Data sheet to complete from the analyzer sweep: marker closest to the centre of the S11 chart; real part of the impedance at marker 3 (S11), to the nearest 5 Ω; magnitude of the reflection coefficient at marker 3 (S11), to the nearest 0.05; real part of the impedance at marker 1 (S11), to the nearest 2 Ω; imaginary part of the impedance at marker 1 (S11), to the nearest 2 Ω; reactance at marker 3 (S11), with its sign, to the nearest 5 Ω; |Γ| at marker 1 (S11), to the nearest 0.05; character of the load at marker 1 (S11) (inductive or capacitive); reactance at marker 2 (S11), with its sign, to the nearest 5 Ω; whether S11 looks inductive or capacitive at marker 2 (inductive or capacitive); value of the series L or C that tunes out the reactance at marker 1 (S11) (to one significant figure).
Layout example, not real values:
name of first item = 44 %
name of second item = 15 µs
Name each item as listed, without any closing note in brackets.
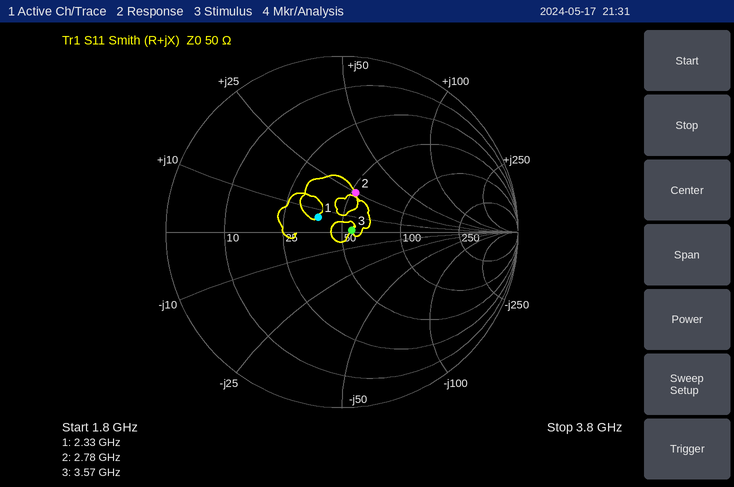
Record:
marker closest to the centre of the S11 chart = marker 3
real part of the impedance at marker 3 (S11), to the nearest 5 Ω = 55 Ω
magnitude of the reflection coefficient at marker 3 (S11), to the nearest 0.05 = 0.05
real part of the impedance at marker 1 (S11), to the nearest 2 Ω = 38 Ω
imaginary part of the impedance at marker 1 (S11), to the nearest 2 Ω = +6 Ω
reactance at marker 3 (S11), with its sign, to the nearest 5 Ω = 0 Ω
|Γ| at marker 1 (S11), to the nearest 0.05 = 0.15
character of the load at marker 1 (S11) = inductive
reactance at marker 2 (S11), with its sign, to the nearest 5 Ω = +25 Ω
whether S11 looks inductive or capacitive at marker 2 = inductive
value of the series L or C that tunes out the reactance at marker 1 (S11) = 10 pF
